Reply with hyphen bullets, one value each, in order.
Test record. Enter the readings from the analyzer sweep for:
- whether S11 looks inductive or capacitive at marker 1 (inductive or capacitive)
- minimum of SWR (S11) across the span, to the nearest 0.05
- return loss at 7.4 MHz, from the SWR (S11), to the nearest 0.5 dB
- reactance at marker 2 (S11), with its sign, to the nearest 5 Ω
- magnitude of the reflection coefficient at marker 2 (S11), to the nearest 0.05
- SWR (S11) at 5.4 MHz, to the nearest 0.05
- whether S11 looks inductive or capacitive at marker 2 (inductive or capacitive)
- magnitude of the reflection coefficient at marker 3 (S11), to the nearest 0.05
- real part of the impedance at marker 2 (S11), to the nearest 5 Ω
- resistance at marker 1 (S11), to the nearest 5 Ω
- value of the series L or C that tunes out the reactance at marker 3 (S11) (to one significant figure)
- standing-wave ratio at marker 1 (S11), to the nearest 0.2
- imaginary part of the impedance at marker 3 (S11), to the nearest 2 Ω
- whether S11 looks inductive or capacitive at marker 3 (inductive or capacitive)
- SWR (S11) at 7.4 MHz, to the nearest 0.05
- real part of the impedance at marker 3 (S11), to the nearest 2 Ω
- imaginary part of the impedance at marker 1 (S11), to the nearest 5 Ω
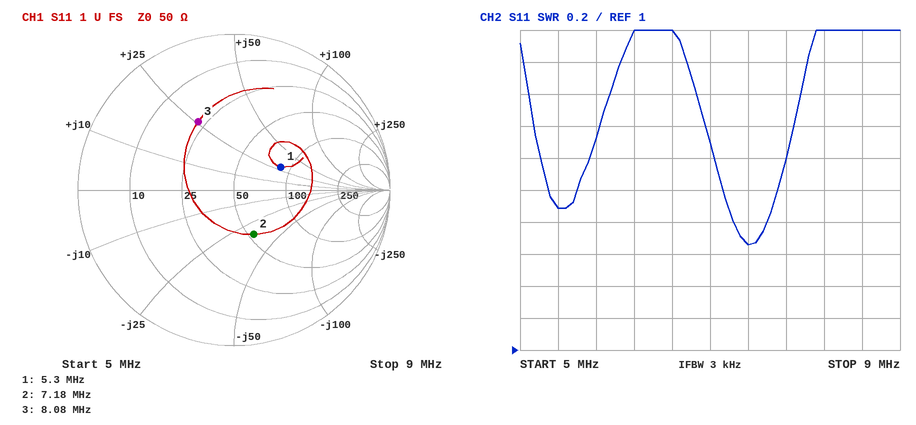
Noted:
- inductive
- 1.65
- 12.0 dB
- -35 Ω
- 0.30
- 1.90
- capacitive
- 0.50
- 55 Ω
- 85 Ω
- 800 pF
- 2.0
- +26 Ω
- inductive
- 1.65
- 22 Ω
- +30 Ω
